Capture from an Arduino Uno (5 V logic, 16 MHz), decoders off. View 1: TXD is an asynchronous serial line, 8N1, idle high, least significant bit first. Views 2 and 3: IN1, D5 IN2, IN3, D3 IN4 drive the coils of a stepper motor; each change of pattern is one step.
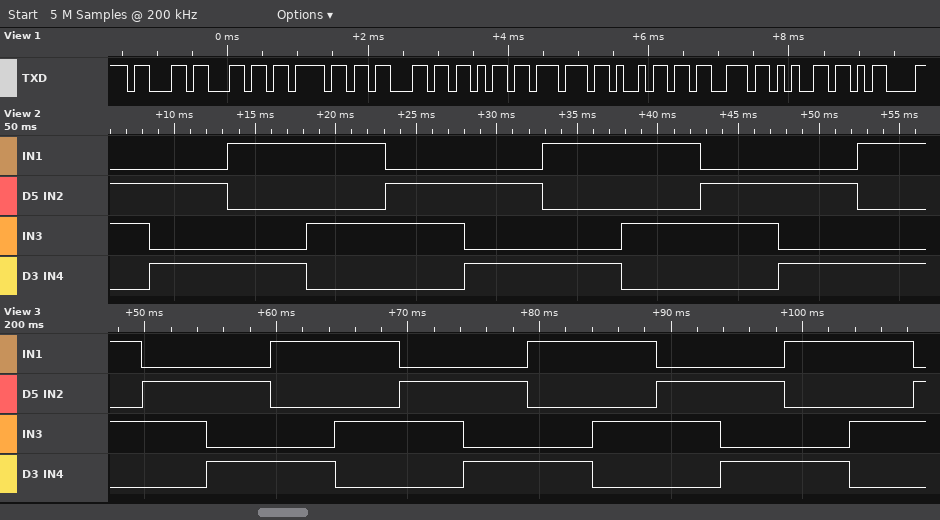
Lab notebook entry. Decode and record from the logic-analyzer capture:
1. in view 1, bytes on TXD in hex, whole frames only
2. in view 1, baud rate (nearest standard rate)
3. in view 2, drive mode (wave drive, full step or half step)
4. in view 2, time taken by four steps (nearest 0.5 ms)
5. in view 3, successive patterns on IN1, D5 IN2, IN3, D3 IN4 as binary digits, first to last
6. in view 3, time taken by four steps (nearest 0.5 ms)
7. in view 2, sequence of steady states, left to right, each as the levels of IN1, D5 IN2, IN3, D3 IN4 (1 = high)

63 6C 6F 63 6B 77 69 73 65 0D
9600 baud
full step
19.5 ms
1010 0110 0101 1001 1010 0110 0101 1001 1010 0110 0101 1001 1010 0110
19.5 ms
0110 0101 1001 1010 0110 0101 1001 1010 0110 0101 1001
